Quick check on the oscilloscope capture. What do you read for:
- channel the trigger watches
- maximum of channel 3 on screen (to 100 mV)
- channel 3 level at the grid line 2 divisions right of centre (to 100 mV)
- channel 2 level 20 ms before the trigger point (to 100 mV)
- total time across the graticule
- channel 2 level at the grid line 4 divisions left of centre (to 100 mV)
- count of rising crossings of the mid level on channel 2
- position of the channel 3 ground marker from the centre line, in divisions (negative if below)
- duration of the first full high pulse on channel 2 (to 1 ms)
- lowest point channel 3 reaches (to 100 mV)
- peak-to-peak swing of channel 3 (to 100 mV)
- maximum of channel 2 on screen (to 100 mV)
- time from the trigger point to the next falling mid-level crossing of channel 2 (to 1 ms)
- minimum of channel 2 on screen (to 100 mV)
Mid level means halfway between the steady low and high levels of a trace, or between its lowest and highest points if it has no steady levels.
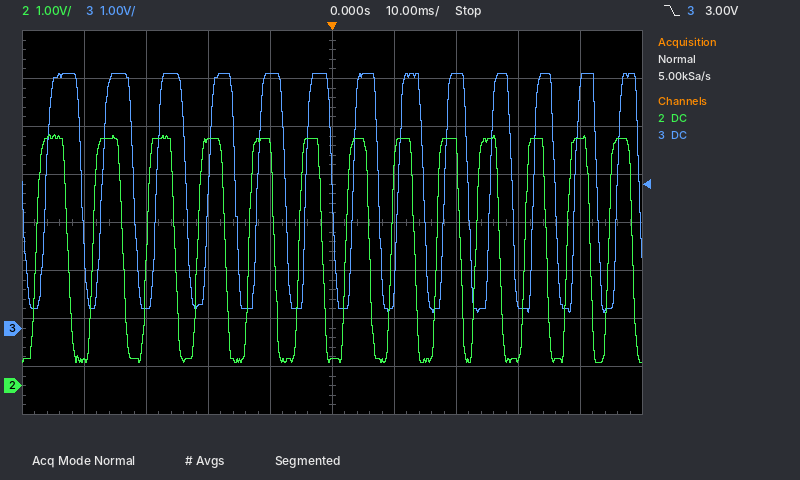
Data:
channel 3
5.3 V
5.3 V
5.1 V
100 ms
500 mV
13
-2.2 div
5 ms
300 mV
5.0 V
5.2 V
6 ms
500 mV
